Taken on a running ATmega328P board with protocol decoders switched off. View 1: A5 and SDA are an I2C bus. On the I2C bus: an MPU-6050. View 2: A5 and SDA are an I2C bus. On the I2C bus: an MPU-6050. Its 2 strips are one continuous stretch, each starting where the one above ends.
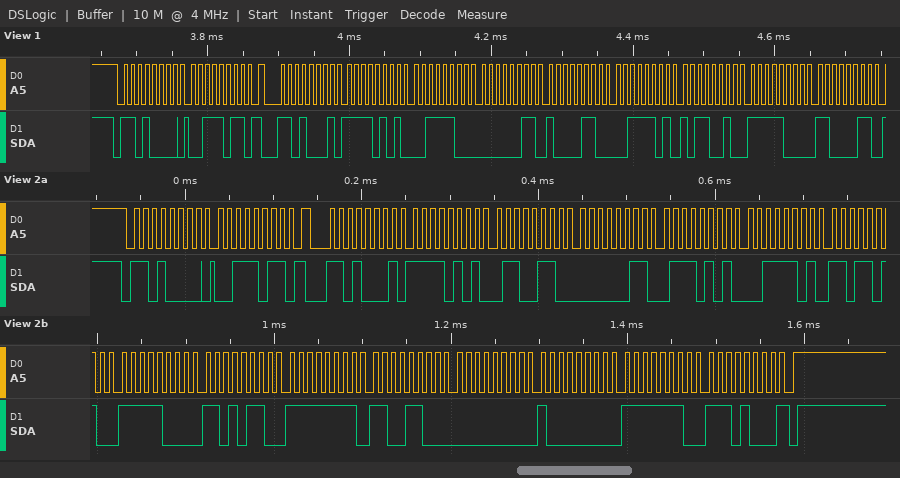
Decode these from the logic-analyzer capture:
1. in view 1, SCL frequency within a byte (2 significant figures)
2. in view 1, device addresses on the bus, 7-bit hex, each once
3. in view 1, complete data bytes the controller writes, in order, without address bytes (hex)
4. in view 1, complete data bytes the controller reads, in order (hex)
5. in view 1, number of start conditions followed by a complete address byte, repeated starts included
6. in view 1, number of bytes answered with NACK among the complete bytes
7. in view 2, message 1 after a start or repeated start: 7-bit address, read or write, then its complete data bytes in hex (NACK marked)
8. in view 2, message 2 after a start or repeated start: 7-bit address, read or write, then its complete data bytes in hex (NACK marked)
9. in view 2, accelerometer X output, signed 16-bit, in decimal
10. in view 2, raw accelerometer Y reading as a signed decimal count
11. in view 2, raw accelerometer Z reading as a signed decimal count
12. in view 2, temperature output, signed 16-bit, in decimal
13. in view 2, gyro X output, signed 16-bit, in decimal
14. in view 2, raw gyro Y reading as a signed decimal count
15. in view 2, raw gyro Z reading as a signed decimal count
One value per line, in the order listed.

100 kHz
0x68
3B
F5 3C 03 86 3D B2 F8 C3
2
0
0x68 write: 3B
0x68 read: F5 66 03 75 3D DA F8 D6 FF CC 00 80 FE E8 NACK
-2714
885
15834
-1834
-52
128
-280
